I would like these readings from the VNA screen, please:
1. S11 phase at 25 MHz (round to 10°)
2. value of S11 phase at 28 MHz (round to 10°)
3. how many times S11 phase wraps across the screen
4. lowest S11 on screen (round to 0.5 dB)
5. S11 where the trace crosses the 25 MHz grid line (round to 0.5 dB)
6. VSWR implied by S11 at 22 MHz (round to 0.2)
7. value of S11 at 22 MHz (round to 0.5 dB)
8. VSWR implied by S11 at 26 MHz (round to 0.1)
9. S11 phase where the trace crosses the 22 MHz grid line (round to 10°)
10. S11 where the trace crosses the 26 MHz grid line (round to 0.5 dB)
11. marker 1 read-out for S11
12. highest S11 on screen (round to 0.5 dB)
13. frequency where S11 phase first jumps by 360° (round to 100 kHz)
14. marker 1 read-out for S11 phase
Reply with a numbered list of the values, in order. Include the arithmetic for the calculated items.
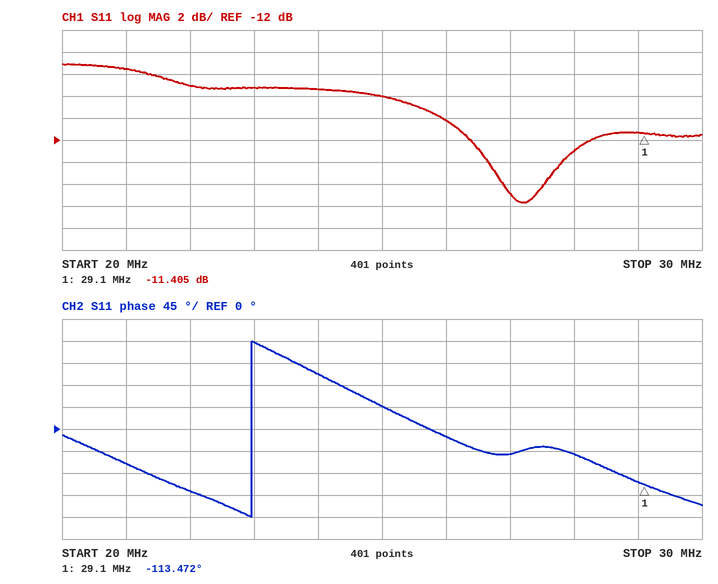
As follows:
1. 50°
2. -50°
3. 1
4. -17.5 dB
5. -8.0 dB
6. |Γ| = 10^(-7/20) = 0.4467; VSWR = (1 + 0.4467)/(1 − 0.4467) ≈ 2.6
7. -7.0 dB
8. |Γ| = 10^(-10/20) = 0.3162; VSWR = (1 + 0.3162)/(1 − 0.3162) ≈ 1.9
9. -130°
10. -10.0 dB
11. -11.405 dB
12. -5.0 dB
13. 23.0 MHz
14. -113.472°
